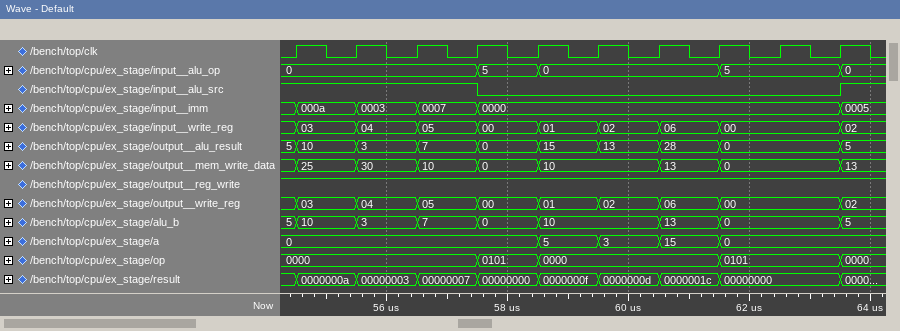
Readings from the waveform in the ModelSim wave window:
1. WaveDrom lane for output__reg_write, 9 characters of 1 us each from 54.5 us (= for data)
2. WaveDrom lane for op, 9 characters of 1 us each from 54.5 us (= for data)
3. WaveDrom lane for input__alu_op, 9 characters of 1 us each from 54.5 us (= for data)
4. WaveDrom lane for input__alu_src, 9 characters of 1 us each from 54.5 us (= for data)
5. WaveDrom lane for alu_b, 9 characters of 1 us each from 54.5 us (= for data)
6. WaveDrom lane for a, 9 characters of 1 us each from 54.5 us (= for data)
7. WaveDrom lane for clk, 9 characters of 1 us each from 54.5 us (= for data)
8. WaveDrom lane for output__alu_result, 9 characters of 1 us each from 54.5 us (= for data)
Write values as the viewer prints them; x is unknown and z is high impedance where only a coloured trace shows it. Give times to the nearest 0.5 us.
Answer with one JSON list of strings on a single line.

["{name: 'output__reg_write', wave: '1........'}", "{name: 'op', wave: '=..==..=.', data: '0000 0101 0000 0101'}", "{name: 'input__alu_op', wave: '=..==..=.', data: '0 5 0 5'}", "{name: 'input__alu_src', wave: '1..0.....'}", "{name: 'alu_b', wave: '=====.==.', data: '10 3 7 0 10 13 0'}", "{name: 'a', wave: '=...====.', data: '0 5 3 15 0'}", "{name: 'clk', wave: 'p........'}", "{name: 'output__alu_result', wave: '========.', data: '10 3 7 0 15 13 28 0'}"]
